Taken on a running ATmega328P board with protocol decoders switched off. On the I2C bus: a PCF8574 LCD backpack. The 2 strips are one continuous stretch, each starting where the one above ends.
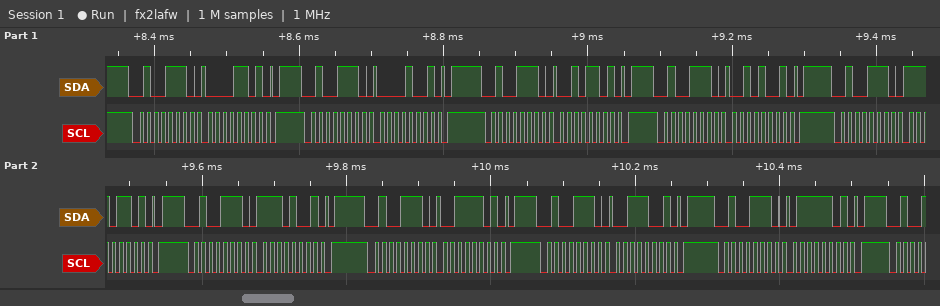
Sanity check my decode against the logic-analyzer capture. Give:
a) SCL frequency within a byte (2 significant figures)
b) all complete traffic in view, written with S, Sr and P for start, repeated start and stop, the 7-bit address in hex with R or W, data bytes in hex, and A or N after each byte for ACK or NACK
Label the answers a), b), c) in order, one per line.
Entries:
a) 100 kHz
b) S 27W A 0D A P S 27W A 09 A P S 27W A 2D A P S 27W A 29 A P S 27W A ED A P S 27W A E9 A P S 27W A 3D A P S 27W A 39 A P S 27W A 7D A P
